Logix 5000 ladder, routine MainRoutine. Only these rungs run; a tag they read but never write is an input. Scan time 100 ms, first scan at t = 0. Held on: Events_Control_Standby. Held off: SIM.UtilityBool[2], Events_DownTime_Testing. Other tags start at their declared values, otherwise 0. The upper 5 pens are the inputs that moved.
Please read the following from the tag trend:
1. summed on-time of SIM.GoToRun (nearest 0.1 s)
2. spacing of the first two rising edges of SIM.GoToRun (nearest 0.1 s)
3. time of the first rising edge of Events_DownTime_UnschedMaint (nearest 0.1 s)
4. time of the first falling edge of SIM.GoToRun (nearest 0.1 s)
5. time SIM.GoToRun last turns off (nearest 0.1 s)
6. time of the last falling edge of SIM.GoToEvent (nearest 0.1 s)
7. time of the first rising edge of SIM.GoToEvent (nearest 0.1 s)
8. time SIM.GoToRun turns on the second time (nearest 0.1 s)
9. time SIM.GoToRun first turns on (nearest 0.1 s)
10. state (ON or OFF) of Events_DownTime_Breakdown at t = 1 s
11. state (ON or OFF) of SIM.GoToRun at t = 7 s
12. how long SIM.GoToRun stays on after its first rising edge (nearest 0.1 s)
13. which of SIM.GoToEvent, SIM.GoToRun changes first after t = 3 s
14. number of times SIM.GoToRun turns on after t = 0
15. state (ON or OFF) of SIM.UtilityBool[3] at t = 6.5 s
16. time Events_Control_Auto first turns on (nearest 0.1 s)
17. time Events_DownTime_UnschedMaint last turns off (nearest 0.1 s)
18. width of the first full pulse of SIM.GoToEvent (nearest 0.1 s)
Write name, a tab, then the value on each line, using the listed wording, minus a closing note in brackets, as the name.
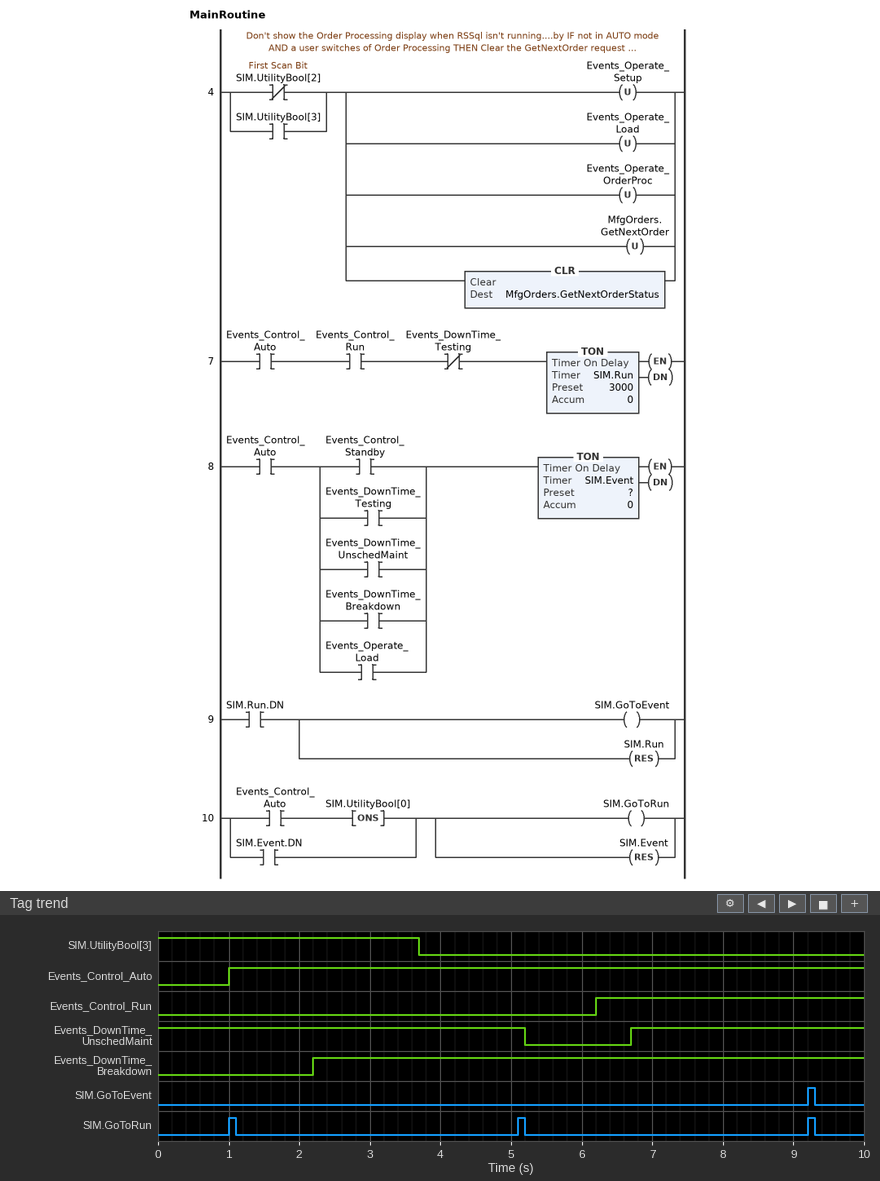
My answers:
summed on-time of SIM.GoToRun	0.3 s
spacing of the first two rising edges of SIM.GoToRun	4.1 s
time of the first rising edge of Events_DownTime_UnschedMaint	6.7 s
time of the first falling edge of SIM.GoToRun	1.1 s
time SIM.GoToRun last turns off	9.3 s
time of the last falling edge of SIM.GoToEvent	9.3 s
time of the first rising edge of SIM.GoToEvent	9.2 s
time SIM.GoToRun turns on the second time	5.1 s
time SIM.GoToRun first turns on	1.0 s
state (ON or OFF) of Events_DownTime_Breakdown at t = 1 s	OFF
state (ON or OFF) of SIM.GoToRun at t = 7 s	OFF
how long SIM.GoToRun stays on after its first rising edge	0.1 s
which of SIM.GoToEvent, SIM.GoToRun changes first after t = 3 s	SIM.GoToRun
number of times SIM.GoToRun turns on after t = 0	3
state (ON or OFF) of SIM.UtilityBool[3] at t = 6.5 s	OFF
time Events_Control_Auto first turns on	1.0 s
time Events_DownTime_UnschedMaint last turns off	5.2 s
width of the first full pulse of SIM.GoToEvent	0.1 s
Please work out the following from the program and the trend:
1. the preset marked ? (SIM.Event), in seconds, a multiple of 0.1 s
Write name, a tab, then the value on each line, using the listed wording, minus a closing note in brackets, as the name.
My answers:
the preset marked ? (SIM.Event), in seconds, a multiple of 0.1 s	4.0 s
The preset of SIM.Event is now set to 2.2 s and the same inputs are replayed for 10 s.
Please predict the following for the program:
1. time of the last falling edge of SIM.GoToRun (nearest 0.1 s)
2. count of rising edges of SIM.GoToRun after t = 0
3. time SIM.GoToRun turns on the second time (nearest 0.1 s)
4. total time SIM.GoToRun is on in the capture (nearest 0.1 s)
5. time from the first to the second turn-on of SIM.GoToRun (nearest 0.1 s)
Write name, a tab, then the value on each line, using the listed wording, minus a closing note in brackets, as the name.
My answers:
time of the last falling edge of SIM.GoToRun	8.0 s
count of rising edges of SIM.GoToRun after t = 0	4
time SIM.GoToRun turns on the second time	3.3 s
total time SIM.GoToRun is on in the capture	0.4 s
time from the first to the second turn-on of SIM.GoToRun	2.3 s
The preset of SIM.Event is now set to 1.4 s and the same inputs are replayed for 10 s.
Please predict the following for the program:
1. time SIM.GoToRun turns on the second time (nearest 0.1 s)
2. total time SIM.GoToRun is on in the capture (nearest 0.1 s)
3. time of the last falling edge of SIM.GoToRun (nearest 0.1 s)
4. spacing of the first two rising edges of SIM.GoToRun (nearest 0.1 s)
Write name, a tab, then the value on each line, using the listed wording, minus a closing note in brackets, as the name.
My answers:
time SIM.GoToRun turns on the second time	2.5 s
total time SIM.GoToRun is on in the capture	0.6 s
time of the last falling edge of SIM.GoToRun	8.6 s
spacing of the first two rising edges of SIM.GoToRun	1.5 s
